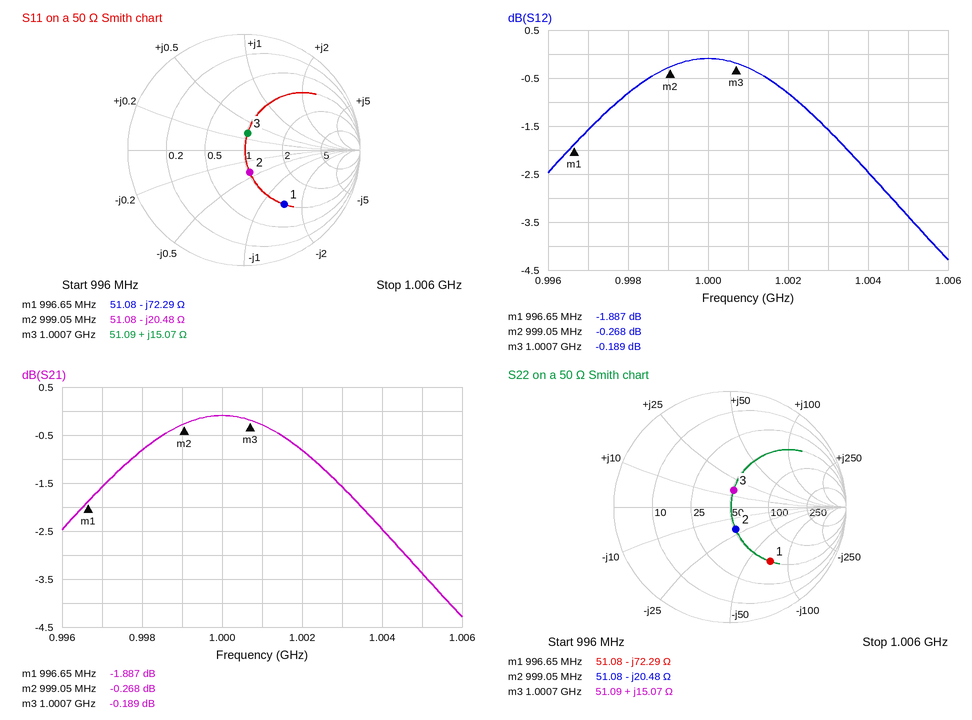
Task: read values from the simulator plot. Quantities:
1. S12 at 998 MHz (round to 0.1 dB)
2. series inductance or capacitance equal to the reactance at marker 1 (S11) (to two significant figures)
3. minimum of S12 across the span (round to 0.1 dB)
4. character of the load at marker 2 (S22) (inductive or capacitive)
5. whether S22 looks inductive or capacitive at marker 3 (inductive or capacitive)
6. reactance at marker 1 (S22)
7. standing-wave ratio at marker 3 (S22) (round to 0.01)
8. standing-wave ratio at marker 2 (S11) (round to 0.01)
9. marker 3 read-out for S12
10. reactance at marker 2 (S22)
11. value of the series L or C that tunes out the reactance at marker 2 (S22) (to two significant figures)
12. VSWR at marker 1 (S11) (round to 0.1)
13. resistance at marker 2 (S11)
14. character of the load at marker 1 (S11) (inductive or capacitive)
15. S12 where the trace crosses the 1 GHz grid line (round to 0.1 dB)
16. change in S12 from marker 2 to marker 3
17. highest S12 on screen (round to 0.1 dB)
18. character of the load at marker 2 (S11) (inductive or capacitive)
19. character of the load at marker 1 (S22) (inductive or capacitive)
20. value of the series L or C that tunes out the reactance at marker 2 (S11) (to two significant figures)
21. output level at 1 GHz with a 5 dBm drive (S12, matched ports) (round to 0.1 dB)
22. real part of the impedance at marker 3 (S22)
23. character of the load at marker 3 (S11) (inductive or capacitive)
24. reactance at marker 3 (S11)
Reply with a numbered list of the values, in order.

1. -0.8 dB
2. 2.2 pF
3. -4.3 dB
4. capacitive
5. inductive
6. -72.29 Ω
7. 1.35
8. 1.50
9. -0.189 dB
10. -20.48 Ω
11. 3.3 nH
12. 3.8
13. 51.08 Ω
14. capacitive
15. -0.1 dB
16. 0.079 dB
17. -0.1 dB
18. capacitive
19. capacitive
20. 3.3 nH
21. 4.9 dBm
22. 51.09 Ω
23. inductive
24. +15.07 Ω
